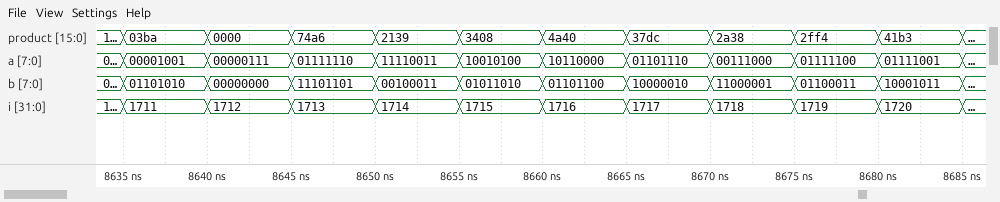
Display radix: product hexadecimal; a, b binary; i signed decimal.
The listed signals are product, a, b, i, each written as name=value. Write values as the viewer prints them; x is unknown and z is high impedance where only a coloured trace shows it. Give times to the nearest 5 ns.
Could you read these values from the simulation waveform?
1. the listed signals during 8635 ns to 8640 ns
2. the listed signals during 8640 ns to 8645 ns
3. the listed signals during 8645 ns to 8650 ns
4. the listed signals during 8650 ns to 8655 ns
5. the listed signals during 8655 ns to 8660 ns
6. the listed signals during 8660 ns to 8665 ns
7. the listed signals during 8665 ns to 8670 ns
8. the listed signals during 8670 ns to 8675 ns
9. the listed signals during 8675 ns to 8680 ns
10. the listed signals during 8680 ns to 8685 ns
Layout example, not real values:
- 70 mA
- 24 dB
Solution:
- product=03ba, a=00001001, b=01101010, i=1711
- product=0000, a=00000111, b=00000000, i=1712
- product=74a6, a=01111110, b=11101101, i=1713
- product=2139, a=11110011, b=00100011, i=1714
- product=3408, a=10010100, b=01011010, i=1715
- product=4a40, a=10110000, b=01101100, i=1716
- product=37dc, a=01101110, b=10000010, i=1717
- product=2a38, a=00111000, b=11000001, i=1718
- product=2ff4, a=01111100, b=01100011, i=1719
- product=41b3, a=01111001, b=10001011, i=1720
